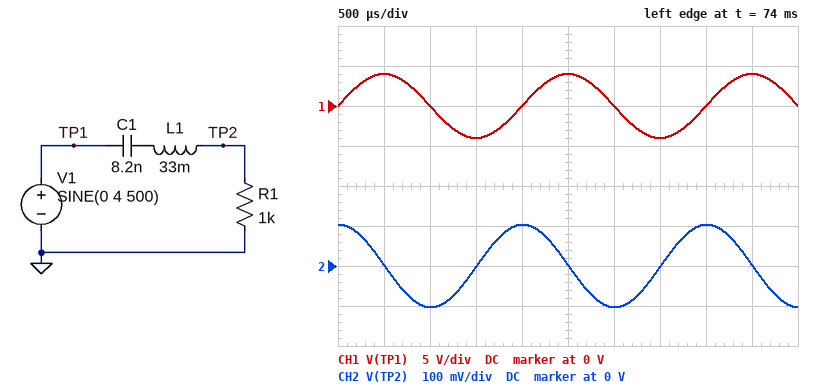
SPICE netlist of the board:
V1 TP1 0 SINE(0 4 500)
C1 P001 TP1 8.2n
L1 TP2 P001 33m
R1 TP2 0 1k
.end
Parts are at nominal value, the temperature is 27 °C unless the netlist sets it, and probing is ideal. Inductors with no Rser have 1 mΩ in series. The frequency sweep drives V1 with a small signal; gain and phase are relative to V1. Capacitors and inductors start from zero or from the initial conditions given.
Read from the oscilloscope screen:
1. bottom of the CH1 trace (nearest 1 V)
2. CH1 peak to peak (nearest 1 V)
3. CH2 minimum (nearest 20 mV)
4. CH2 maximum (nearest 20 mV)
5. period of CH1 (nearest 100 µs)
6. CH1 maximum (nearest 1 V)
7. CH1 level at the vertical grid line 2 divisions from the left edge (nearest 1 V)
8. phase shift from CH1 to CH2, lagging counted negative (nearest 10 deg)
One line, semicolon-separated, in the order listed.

-4 V; 8 V; -100 mV; 100 mV; 2.0 ms; 4 V; 0 V; 90 deg
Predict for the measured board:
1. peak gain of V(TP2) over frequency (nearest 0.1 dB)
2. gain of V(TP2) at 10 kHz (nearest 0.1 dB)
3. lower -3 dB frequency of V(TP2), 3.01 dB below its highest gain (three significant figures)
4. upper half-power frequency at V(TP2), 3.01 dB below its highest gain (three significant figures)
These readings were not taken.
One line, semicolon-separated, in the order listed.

0 dB; -0.1 dB; 7.56 kHz; 12.4 kHz
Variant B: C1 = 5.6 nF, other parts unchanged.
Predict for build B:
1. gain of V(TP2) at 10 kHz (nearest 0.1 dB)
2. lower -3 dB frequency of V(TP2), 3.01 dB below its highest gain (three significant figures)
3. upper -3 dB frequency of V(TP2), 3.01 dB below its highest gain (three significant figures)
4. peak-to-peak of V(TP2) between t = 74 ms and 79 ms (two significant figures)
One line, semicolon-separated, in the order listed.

-2.0 dB; 9.54 kHz; 14.4 kHz; 140 mV
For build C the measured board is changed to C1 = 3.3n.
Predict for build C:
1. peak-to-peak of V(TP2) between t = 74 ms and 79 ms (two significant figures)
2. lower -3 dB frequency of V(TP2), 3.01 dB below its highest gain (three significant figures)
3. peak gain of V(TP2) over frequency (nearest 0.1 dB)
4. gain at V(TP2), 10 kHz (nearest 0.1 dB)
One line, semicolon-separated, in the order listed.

83 mV; 13.0 kHz; 0 dB; -9.3 dB
